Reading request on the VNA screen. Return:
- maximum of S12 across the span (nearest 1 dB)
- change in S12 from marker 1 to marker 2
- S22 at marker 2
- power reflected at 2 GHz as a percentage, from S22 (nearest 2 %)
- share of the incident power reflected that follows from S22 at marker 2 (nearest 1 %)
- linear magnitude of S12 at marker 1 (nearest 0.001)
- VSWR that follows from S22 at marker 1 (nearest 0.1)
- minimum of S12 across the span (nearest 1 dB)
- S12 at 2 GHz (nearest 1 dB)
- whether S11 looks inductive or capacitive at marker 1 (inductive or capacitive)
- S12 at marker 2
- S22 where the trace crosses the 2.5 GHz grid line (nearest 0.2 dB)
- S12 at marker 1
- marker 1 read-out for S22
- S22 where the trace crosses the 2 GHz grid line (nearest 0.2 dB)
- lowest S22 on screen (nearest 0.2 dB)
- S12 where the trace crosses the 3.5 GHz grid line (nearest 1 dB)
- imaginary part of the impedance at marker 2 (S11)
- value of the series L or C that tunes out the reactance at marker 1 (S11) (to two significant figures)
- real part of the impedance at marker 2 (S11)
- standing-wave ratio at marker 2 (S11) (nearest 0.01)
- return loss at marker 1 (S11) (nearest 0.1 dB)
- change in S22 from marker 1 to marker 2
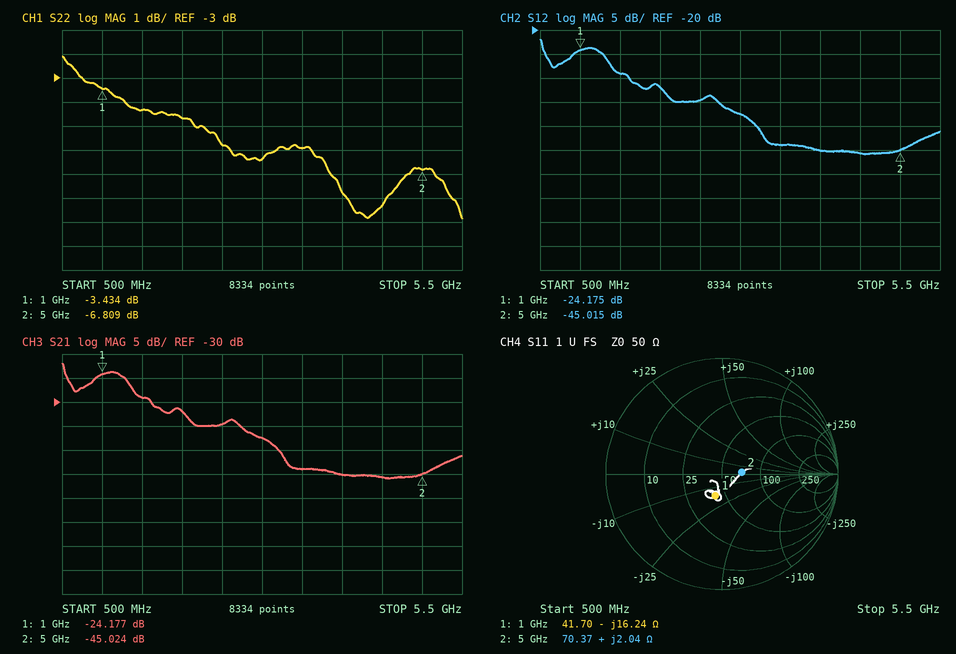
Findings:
-22 dB
-20.840 dB
-6.809 dB
34 %
21 %
0.062
5.1
-46 dB
-32 dB
capacitive
-45.015 dB
-5.8 dB
-24.175 dB
-3.434 dB
-4.6 dB
-8.8 dB
-44 dB
+2.04 Ω
2.6 nH
70.37 Ω
1.41
14.2 dB
-3.375 dB
